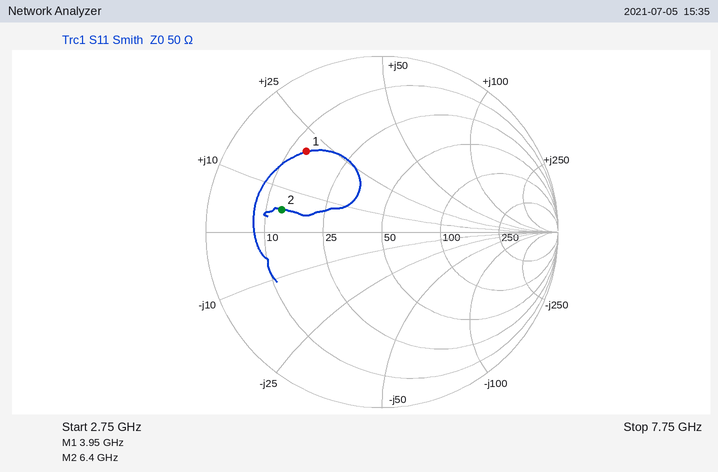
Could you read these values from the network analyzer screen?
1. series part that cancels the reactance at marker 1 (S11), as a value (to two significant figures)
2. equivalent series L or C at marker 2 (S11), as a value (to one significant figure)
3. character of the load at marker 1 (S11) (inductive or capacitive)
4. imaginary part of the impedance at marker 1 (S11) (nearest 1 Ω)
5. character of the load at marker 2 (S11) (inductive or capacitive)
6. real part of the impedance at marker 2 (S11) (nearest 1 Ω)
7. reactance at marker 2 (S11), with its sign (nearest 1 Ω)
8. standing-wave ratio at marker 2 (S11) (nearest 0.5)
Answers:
2.0 pF
100 pH
inductive
+20 Ω
inductive
13 Ω
+5 Ω
4.0
